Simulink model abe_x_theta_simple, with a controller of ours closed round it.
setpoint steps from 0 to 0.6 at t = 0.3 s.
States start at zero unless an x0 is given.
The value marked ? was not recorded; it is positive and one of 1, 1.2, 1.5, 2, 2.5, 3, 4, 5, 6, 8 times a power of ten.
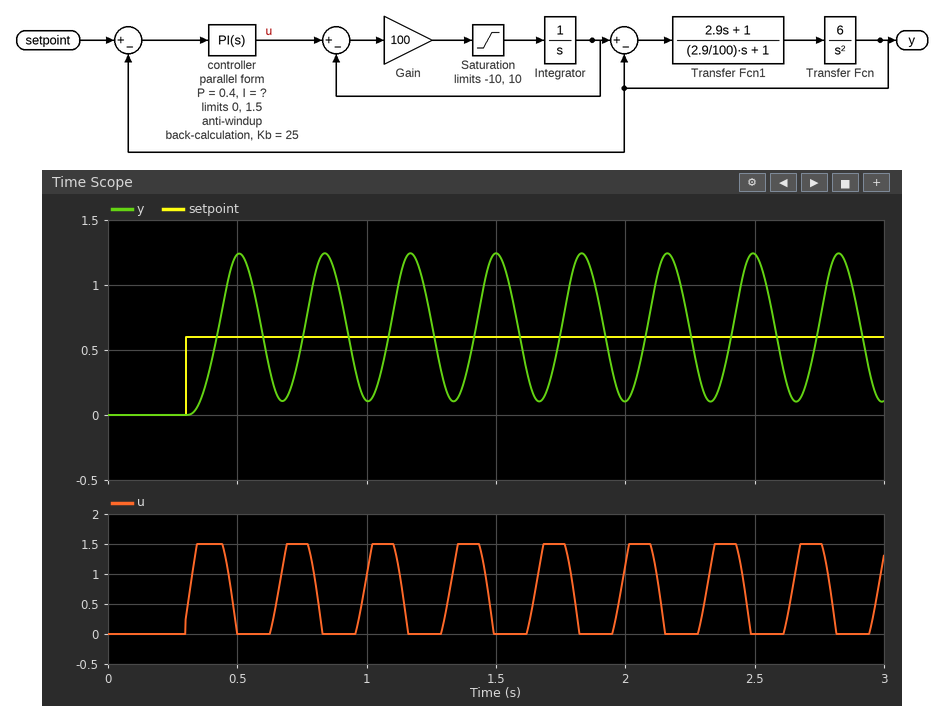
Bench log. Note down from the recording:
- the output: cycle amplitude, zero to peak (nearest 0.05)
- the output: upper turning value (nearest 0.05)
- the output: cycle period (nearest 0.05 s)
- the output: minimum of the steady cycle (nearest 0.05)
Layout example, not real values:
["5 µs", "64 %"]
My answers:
["0.55", "1.25", "0.35 s", "0.10"]
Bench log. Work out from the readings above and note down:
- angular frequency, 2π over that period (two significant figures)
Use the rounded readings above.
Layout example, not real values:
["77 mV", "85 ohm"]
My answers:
["18 rad/s"]
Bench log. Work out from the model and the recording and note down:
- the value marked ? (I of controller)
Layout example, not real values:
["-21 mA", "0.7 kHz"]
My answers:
["50"]
